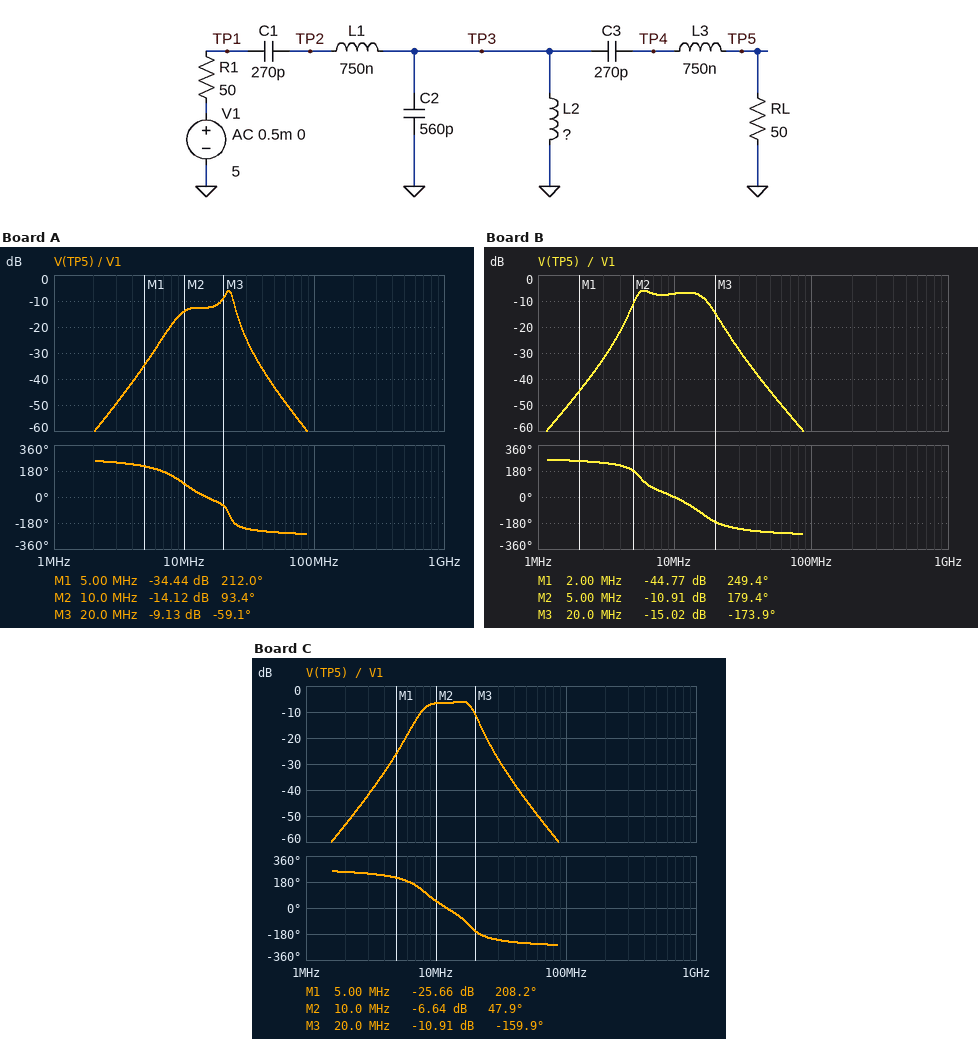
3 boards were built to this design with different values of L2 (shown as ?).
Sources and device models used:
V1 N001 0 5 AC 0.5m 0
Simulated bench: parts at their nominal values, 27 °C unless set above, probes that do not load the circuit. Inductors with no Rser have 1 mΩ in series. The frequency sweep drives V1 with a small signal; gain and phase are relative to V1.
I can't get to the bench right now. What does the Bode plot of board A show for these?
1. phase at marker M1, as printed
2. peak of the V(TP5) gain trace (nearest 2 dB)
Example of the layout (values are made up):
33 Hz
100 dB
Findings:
212.0 deg
-6 dB
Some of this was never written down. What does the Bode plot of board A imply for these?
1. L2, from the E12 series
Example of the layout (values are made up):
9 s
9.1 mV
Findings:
120 nH
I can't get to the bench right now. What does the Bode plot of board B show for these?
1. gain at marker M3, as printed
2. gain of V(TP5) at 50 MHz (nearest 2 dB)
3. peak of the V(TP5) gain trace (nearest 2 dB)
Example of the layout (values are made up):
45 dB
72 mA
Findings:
-15.02 dB
-44 dB
-6 dB
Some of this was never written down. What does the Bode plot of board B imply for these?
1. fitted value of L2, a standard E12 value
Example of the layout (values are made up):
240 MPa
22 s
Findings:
680 nH
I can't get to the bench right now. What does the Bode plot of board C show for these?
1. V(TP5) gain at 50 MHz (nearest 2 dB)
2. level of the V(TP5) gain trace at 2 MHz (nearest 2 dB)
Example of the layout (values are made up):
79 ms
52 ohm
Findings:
-44 dB
-54 dB
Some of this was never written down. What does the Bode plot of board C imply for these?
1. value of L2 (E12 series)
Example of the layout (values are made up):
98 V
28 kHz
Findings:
270 nH
